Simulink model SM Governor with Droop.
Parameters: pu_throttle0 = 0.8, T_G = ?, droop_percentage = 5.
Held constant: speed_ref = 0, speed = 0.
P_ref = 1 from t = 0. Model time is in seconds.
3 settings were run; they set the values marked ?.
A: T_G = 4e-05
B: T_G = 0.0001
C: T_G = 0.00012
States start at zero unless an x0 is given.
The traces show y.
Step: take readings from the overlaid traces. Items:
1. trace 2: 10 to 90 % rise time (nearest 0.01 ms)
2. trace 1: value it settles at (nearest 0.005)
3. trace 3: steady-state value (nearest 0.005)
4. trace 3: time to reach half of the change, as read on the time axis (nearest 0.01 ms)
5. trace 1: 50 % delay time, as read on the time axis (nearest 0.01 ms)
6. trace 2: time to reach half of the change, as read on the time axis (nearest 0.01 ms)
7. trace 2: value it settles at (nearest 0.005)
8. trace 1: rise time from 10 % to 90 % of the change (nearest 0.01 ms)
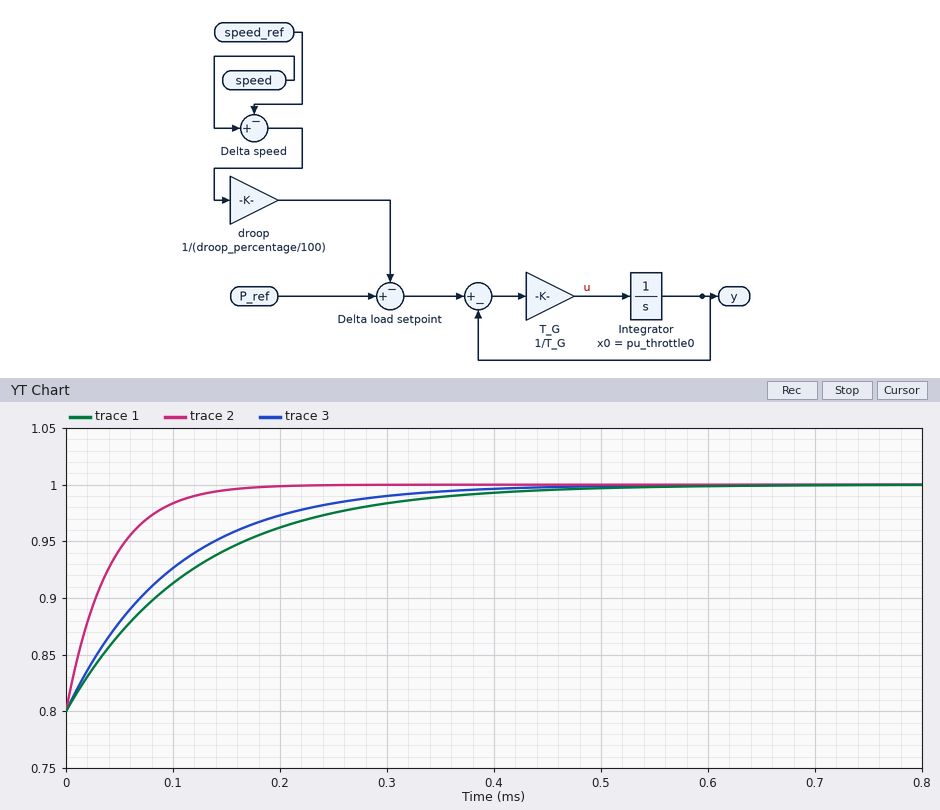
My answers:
0.09 ms
1.000
1.000
0.07 ms
0.08 ms
0.03 ms
1.000
0.26 ms
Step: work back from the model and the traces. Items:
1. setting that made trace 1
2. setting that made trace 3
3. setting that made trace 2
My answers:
C
B
A
